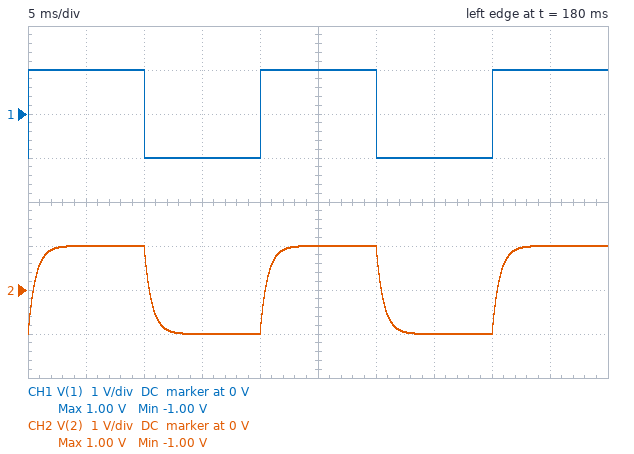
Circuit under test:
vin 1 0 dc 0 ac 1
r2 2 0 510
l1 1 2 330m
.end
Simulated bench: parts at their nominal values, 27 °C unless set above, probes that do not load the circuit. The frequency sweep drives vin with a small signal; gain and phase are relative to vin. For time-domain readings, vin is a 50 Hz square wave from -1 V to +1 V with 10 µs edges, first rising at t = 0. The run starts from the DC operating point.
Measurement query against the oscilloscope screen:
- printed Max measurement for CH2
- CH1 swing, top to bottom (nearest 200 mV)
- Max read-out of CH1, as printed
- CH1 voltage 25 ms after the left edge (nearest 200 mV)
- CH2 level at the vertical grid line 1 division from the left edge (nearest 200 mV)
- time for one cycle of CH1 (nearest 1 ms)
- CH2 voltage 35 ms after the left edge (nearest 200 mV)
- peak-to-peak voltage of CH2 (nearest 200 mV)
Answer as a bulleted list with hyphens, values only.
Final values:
- 1.00 V
- 2.0 V
- 1.00 V
- 1.0 V
- 1.0 V
- 20 ms
- -1.0 V
- 2.0 V
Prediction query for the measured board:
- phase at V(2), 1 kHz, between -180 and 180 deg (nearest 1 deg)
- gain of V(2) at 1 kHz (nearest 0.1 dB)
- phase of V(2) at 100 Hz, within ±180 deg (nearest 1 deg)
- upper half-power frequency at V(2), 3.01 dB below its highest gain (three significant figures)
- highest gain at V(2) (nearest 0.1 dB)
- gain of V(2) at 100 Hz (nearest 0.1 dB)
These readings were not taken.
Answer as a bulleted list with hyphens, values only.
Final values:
- -76 deg
- -12.4 dB
- -22 deg
- 246 Hz
- 0 dB
- -0.7 dB
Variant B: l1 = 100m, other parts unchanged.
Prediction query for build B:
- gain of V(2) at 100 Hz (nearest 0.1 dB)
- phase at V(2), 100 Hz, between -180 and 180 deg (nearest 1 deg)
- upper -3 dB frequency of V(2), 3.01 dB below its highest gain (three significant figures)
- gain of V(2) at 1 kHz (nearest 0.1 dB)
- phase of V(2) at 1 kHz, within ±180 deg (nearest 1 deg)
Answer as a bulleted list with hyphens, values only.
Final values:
- -0.1 dB
- -7 deg
- 812 Hz
- -4.0 dB
- -51 deg
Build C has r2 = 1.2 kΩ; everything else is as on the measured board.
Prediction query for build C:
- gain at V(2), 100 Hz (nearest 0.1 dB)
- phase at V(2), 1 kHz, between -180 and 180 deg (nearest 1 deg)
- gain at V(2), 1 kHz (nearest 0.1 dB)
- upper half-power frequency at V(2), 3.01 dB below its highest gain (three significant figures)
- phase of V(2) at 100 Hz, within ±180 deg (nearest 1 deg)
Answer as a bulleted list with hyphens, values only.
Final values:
- -0.1 dB
- -60 deg
- -6.0 dB
- 579 Hz
- -10 deg
